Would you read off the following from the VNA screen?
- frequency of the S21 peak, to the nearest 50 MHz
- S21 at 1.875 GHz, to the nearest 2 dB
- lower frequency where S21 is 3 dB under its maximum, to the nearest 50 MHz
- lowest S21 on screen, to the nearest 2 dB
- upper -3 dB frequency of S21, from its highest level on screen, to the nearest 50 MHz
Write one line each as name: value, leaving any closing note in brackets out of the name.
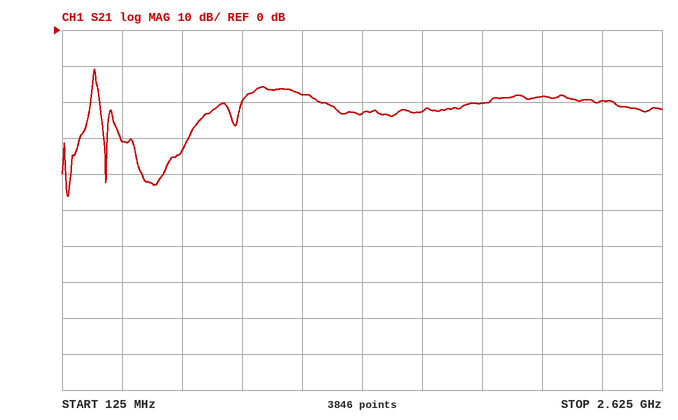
frequency of the S21 peak, to the nearest 50 MHz: 250 MHz
S21 at 1.875 GHz, to the nearest 2 dB: -20 dB
lower frequency where S21 is 3 dB under its maximum, to the nearest 50 MHz: 250 MHz
lowest S21 on screen, to the nearest 2 dB: -46 dB
upper -3 dB frequency of S21, from its highest level on screen, to the nearest 50 MHz: 250 MHz
